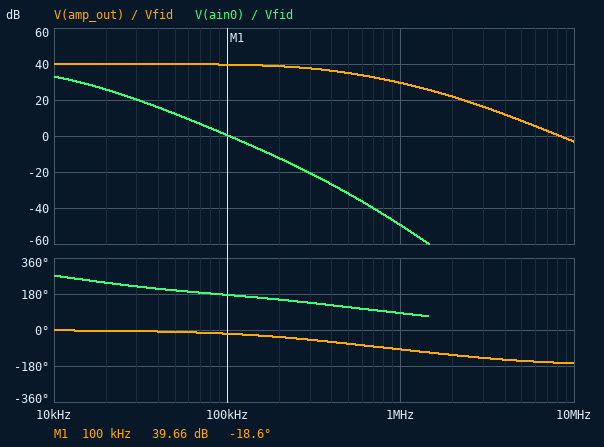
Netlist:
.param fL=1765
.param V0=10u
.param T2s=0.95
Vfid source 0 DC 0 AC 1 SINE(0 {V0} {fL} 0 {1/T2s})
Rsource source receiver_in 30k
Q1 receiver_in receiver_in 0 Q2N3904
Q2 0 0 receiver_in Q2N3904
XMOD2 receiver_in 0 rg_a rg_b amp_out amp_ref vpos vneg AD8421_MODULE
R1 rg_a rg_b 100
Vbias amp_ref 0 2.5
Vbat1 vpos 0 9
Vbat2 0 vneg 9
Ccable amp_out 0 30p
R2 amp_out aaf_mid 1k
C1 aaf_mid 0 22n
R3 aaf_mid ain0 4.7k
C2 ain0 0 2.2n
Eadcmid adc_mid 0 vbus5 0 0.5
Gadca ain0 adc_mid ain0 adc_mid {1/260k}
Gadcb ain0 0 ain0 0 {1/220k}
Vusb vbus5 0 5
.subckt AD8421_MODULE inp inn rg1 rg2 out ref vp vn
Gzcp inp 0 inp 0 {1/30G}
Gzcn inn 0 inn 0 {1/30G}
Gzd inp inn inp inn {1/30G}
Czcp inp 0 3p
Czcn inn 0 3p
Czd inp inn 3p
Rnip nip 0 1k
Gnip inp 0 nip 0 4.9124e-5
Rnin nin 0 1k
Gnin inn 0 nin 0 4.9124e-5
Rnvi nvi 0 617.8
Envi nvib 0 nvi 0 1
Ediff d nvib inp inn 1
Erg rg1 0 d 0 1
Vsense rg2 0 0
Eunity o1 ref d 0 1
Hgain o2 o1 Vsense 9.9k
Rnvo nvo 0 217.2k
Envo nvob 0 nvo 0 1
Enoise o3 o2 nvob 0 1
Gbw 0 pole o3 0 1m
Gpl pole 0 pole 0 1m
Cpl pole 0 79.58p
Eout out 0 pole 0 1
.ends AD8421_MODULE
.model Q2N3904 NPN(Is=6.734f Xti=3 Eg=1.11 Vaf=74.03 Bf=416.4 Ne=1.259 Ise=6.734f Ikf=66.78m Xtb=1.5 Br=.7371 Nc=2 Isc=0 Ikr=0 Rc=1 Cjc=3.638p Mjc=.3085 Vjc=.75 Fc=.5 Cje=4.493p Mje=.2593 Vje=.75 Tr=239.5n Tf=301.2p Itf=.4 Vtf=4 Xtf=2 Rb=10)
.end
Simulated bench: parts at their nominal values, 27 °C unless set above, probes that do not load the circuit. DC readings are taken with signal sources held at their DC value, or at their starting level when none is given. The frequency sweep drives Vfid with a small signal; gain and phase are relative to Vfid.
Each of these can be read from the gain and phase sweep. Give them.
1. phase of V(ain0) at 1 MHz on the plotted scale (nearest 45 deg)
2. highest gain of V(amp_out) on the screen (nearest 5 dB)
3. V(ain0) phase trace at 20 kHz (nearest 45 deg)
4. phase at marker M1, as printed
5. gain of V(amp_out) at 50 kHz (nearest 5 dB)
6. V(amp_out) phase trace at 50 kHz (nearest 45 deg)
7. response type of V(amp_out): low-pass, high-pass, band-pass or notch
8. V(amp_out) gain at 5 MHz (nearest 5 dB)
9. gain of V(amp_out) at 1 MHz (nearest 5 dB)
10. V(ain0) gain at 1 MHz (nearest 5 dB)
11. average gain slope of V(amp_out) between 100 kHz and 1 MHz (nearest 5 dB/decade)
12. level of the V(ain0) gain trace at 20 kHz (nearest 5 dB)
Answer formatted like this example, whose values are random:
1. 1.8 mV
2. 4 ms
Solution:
1. 90 deg
2. 40 dB
3. 225 deg
4. -18.6 deg
5. 40 dB
6. 0 deg
7. low-pass
8. 10 dB
9. 30 dB
10. -50 dB
11. -10 dB/decade
12. 25 dB
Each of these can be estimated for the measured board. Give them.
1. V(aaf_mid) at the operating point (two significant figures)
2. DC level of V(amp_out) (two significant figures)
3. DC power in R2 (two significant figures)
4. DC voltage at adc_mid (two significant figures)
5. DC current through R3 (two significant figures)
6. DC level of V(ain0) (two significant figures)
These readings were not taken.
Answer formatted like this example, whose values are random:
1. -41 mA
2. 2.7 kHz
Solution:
1. 2.5 V
2. 2.5 V
3. 120 nW
4. 2.5 V
5. 11 µA
6. 2.4 V
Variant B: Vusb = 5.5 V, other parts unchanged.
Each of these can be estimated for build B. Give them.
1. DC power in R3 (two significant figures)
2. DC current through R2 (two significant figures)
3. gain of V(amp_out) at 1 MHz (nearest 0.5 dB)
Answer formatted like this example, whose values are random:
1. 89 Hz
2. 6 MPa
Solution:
1. 460 nW
2. 9.9 µA
3. 29.5 dB
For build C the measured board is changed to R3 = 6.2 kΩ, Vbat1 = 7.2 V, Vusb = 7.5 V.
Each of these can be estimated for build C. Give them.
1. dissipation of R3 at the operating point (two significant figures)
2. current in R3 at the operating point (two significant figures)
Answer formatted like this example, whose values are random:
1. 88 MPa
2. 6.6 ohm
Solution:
1. 240 nW
2. 6.2 µA
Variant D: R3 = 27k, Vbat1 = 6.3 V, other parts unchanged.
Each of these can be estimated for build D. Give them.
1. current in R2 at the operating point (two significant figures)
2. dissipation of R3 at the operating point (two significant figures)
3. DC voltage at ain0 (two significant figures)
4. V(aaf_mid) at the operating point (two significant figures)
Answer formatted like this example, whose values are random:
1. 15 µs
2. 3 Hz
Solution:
1. 9.2 µA
2. 2.3 µW
3. 2.2 V
4. 2.5 V
